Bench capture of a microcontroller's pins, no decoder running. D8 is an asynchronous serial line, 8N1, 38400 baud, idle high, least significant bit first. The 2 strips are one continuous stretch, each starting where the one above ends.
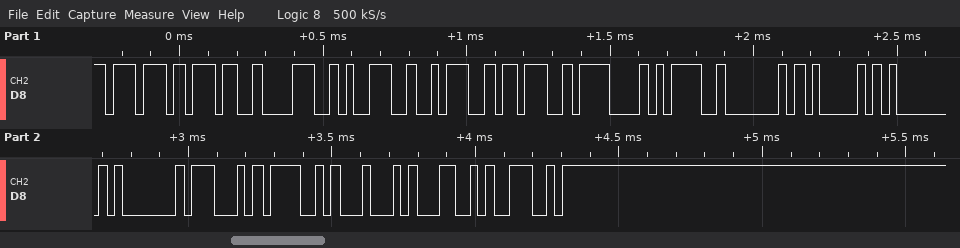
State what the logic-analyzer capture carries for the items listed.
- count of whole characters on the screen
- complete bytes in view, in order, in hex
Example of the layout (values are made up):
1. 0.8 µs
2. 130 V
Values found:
1. 17
2. 0x77 0x37 0x38 0x39 0x3A 0x3B 0x0F 0x3D 0x40 0x41 0x01 0x01 0x47 0x4F 0x44 0x4C 0x4E
